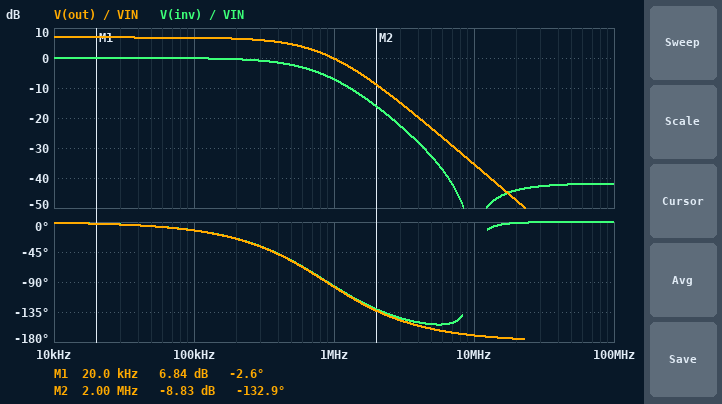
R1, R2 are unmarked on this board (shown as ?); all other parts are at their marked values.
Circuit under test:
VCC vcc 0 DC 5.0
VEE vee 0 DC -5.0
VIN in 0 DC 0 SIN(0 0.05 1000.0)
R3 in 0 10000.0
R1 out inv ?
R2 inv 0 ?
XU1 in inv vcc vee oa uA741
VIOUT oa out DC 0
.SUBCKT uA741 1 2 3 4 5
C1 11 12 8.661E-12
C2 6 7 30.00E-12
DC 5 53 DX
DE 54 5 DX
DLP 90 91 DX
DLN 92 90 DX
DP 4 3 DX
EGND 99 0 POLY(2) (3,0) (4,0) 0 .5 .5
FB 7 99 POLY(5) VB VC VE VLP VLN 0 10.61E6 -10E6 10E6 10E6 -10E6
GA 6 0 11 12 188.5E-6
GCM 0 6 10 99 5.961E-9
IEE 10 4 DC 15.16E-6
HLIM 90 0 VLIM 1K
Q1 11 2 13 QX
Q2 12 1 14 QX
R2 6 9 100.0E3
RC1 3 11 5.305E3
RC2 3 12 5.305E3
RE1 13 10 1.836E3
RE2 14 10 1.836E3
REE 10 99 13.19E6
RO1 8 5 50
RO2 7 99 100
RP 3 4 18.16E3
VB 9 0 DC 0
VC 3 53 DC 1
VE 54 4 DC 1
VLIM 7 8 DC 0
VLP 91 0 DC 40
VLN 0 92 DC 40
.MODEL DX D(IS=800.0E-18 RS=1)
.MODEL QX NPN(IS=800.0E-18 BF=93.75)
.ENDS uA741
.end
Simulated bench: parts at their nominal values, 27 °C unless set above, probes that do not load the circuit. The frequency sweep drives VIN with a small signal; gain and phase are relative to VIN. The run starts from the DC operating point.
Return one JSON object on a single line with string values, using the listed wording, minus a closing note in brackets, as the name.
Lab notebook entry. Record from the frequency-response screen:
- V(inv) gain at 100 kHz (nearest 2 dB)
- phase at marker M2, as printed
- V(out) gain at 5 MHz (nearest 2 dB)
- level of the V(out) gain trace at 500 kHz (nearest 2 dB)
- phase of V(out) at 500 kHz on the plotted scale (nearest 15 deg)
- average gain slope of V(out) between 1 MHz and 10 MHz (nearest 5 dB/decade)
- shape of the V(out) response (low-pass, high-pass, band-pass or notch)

{"V(inv) gain at 100 kHz": "0 dB", "phase at marker M2, as printed": "-132.9 deg", "V(out) gain at 5 MHz": "-24 dB", "level of the V(out) gain trace at 500 kHz": "4 dB", "phase of V(out) at 500 kHz on the plotted scale": "-60 deg", "average gain slope of V(out) between 1 MHz and 10 MHz": "-35 dB/decade", "shape of the V(out) response": "low-pass"}
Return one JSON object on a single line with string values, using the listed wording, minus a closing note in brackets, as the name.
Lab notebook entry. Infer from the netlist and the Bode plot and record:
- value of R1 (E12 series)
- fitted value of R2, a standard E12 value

{"value of R1": "18 kΩ", "fitted value of R2, a standard E12 value": "15 kΩ"}
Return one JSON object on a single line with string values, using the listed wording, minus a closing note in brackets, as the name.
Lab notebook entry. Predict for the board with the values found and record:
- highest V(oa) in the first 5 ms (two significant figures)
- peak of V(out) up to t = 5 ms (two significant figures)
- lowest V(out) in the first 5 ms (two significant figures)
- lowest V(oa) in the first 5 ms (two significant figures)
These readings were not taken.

{"highest V(oa) in the first 5 ms": "110 mV", "peak of V(out) up to t = 5 ms": "110 mV", "lowest V(out) in the first 5 ms": "-110 mV", "lowest V(oa) in the first 5 ms": "-110 mV"}
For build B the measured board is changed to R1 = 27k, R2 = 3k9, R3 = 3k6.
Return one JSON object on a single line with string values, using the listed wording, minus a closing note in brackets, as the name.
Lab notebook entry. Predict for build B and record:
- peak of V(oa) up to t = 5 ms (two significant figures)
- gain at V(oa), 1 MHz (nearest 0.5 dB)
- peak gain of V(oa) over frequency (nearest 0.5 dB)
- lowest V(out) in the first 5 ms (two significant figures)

{"peak of V(oa) up to t = 5 ms": "400 mV", "gain at V(oa), 1 MHz": "-1.0 dB", "peak gain of V(oa) over frequency": "18.0 dB", "lowest V(out) in the first 5 ms": "-390 mV"}
